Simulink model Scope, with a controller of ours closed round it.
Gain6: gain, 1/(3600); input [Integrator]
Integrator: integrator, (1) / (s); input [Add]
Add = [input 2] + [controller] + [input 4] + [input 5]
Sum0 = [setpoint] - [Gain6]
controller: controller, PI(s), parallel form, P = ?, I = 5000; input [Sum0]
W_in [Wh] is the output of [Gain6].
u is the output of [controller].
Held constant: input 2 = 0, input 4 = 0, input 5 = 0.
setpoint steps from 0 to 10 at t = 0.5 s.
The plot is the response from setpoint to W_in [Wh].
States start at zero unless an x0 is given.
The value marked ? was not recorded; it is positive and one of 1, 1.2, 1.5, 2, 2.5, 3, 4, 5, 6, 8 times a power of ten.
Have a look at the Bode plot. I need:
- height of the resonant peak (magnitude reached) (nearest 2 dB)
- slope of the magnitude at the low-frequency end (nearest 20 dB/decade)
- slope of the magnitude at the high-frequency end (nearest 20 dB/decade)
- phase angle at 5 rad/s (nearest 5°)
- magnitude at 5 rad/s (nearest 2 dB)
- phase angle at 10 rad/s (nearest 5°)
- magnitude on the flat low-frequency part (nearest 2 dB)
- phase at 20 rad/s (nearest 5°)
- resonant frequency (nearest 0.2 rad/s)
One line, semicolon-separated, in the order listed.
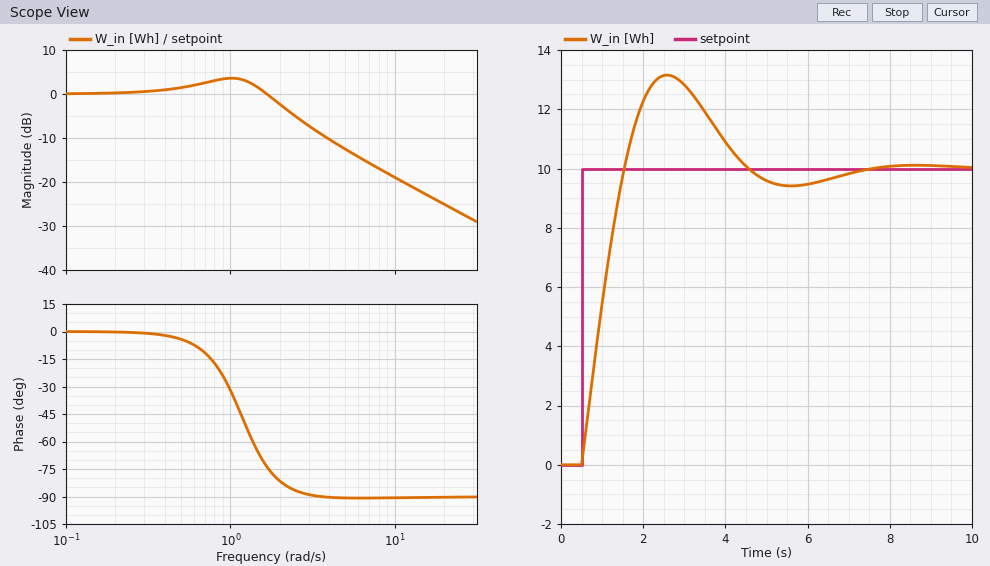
4 dB; 0 dB/decade; -20 dB/decade; -90°; -12 dB; -90°; 0 dB; -90°; 1.0 rad/s
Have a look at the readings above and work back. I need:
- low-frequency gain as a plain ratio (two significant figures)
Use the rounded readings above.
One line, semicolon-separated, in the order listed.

1.0
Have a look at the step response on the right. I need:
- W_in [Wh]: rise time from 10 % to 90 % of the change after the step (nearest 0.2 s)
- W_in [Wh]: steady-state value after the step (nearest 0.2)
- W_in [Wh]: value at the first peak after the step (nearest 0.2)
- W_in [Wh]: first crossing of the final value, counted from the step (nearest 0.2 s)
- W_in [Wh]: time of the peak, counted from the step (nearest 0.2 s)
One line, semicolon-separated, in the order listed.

0.8 s; 10.0; 13.2; 1.0 s; 2.0 s
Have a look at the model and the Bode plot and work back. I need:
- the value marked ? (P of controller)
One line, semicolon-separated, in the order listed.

4000
